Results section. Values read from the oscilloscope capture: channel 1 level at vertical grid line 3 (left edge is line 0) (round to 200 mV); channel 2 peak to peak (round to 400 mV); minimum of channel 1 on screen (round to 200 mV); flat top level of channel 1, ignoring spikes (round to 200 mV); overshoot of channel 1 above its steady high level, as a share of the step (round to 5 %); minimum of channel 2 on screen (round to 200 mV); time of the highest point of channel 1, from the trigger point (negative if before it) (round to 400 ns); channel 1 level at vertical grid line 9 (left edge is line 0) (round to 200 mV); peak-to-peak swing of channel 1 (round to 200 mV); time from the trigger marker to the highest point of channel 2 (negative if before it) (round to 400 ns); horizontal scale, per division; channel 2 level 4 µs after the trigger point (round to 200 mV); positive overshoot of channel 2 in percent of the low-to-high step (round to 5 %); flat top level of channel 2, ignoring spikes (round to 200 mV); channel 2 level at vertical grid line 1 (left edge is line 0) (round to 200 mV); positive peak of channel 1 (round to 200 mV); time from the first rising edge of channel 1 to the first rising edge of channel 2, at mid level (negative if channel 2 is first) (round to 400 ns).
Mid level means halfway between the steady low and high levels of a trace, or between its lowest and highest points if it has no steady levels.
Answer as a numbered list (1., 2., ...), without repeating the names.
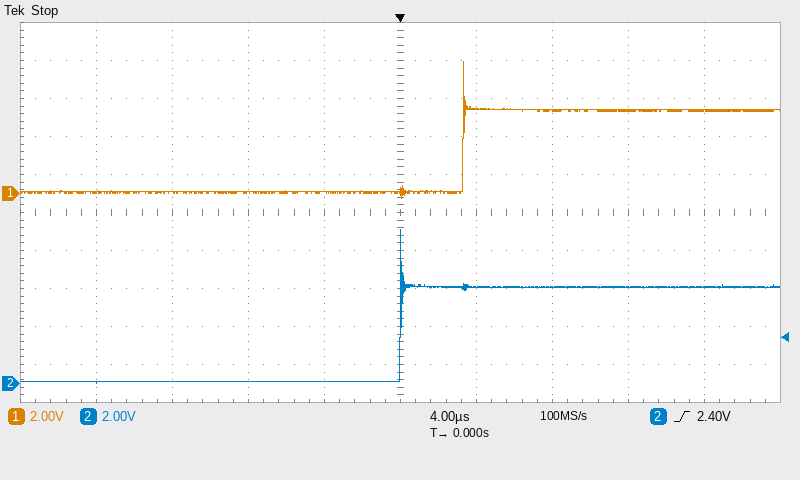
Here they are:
1. 0.0 V
2. 8.0 V
3. -200 mV
4. 4.4 V
5. 60 %
6. 0.0 V
7. +3.2 µs
8. 4.4 V
9. 7.2 V
10. 0.0 µs
11. 4 µs
12. 5.0 V
13. 60 %
14. 5.0 V
15. 0.0 V
16. 7.0 V
17. -3.2 µs
